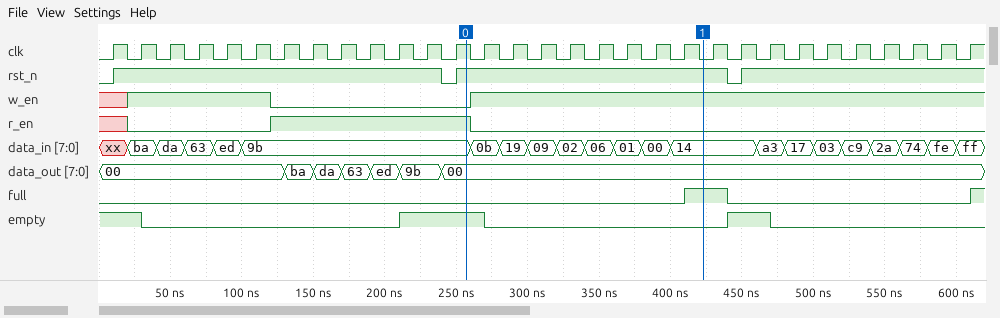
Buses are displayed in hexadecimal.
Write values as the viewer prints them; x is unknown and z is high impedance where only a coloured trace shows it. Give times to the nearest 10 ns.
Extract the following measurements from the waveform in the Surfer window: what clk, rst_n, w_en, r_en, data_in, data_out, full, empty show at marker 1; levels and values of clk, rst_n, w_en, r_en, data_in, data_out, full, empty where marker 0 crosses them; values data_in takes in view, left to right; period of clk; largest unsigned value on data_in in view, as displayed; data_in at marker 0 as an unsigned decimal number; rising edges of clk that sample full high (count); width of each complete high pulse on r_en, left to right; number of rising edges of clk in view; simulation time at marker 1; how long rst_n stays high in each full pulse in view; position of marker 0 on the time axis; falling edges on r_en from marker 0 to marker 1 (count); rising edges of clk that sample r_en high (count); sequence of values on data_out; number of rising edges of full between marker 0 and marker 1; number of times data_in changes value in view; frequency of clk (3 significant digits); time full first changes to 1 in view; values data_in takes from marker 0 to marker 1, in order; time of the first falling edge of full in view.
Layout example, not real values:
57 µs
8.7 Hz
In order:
clk=0, rst_n=1, w_en=1, r_en=0, data_in=14, data_out=00, full=1, empty=0
clk=1, rst_n=1, w_en=0, r_en=1, data_in=9b, data_out=00, full=0, empty=1
xx, ba, da, 63, ed, 9b, 0b, 19, 09, 02, 06, 01, 00, 14, a3, 17, 03, c9, 2a, 74, fe, ff
20 ns
ff
155
1
140 ns
31
420 ns
230 ns, 190 ns
260 ns
1
7
00, ba, da, 63, ed, 9b, 00
1
21
50.0 MHz
410 ns
9b, 0b, 19, 09, 02, 06, 01, 00, 14
440 ns
